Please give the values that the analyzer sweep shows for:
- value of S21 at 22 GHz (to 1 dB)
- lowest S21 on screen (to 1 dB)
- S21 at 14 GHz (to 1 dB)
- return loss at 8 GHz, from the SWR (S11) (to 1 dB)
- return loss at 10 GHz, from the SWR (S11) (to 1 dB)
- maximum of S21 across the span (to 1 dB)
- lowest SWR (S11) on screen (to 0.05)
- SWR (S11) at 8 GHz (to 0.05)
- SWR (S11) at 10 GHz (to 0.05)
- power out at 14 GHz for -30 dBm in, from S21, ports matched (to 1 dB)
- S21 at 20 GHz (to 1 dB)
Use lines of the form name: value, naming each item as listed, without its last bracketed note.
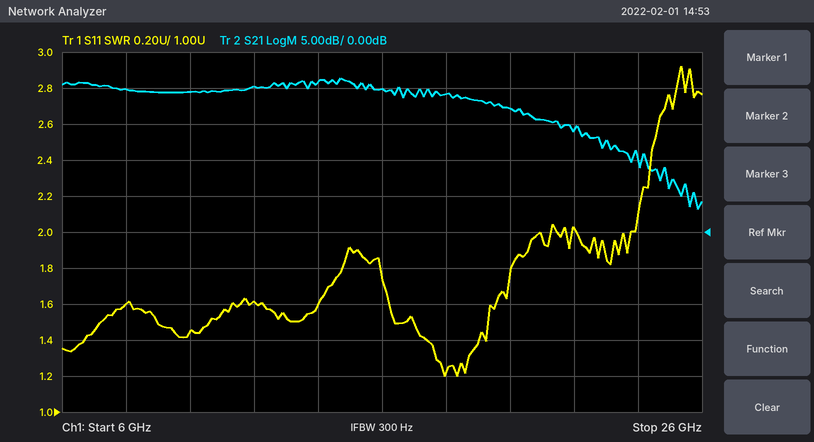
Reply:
value of S21 at 22 GHz: 14 dB
lowest S21 on screen: 3 dB
S21 at 14 GHz: 21 dB
return loss at 8 GHz, from the SWR (S11): 13 dB
return loss at 10 GHz, from the SWR (S11): 15 dB
maximum of S21 across the span: 21 dB
lowest SWR (S11) on screen: 1.20
SWR (S11) at 8 GHz: 1.60
SWR (S11) at 10 GHz: 1.45
power out at 14 GHz for -30 dBm in, from S21, ports matched: -9 dBm
S21 at 20 GHz: 17 dB
